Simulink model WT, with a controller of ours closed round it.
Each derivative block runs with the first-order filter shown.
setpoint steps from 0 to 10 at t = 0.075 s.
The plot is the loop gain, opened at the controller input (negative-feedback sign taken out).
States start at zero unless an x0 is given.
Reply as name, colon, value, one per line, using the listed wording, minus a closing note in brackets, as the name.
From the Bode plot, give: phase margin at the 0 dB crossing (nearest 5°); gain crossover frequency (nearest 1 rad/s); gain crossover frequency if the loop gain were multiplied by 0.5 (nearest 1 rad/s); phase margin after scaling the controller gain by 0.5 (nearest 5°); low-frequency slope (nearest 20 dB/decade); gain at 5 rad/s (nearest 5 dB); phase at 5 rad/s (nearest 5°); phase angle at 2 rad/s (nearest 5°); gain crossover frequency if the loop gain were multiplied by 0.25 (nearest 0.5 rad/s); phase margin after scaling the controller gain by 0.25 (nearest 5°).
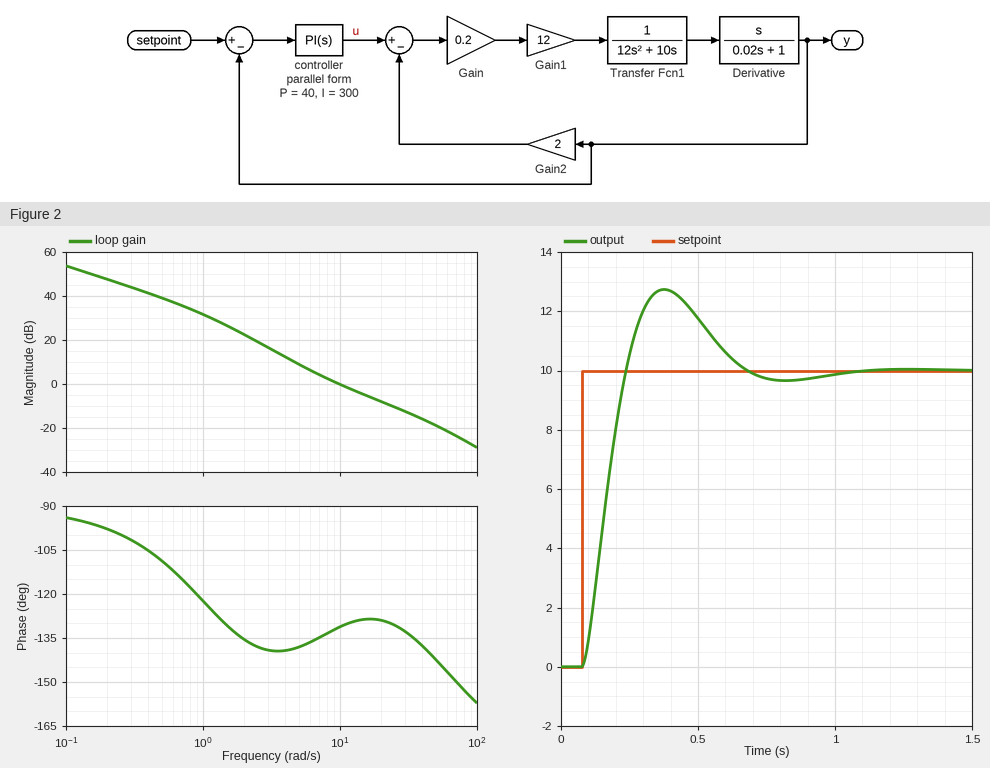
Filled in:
phase margin at the 0 dB crossing: 50°
gain crossover frequency: 10 rad/s
gain crossover frequency if the loop gain were multiplied by 0.5: 6 rad/s
phase margin after scaling the controller gain by 0.5: 45°
low-frequency slope: -20 dB/decade
gain at 5 rad/s: 10 dB
phase at 5 rad/s: -140°
phase angle at 2 rad/s: -135°
gain crossover frequency if the loop gain were multiplied by 0.25: 4.0 rad/s
phase margin after scaling the controller gain by 0.25: 40°
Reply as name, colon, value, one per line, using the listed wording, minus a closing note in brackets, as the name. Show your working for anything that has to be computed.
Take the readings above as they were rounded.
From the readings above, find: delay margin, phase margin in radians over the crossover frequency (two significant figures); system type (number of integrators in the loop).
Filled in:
delay margin, phase margin in radians over the crossover frequency: 50 × π / 180 / 10 = 0.087 s
system type: 1
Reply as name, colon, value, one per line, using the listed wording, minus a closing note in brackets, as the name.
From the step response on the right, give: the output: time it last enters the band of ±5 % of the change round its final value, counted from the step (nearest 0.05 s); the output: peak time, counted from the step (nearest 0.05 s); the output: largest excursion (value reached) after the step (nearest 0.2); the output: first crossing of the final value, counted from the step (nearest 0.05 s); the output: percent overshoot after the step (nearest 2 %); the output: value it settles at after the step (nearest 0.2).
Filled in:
the output: time it last enters the band of ±5 % of the change round its final value, counted from the step: 0.55 s
the output: peak time, counted from the step: 0.30 s
the output: largest excursion (value reached) after the step: 12.8
the output: first crossing of the final value, counted from the step: 0.15 s
the output: percent overshoot after the step: 28 %
the output: value it settles at after the step: 10.0
